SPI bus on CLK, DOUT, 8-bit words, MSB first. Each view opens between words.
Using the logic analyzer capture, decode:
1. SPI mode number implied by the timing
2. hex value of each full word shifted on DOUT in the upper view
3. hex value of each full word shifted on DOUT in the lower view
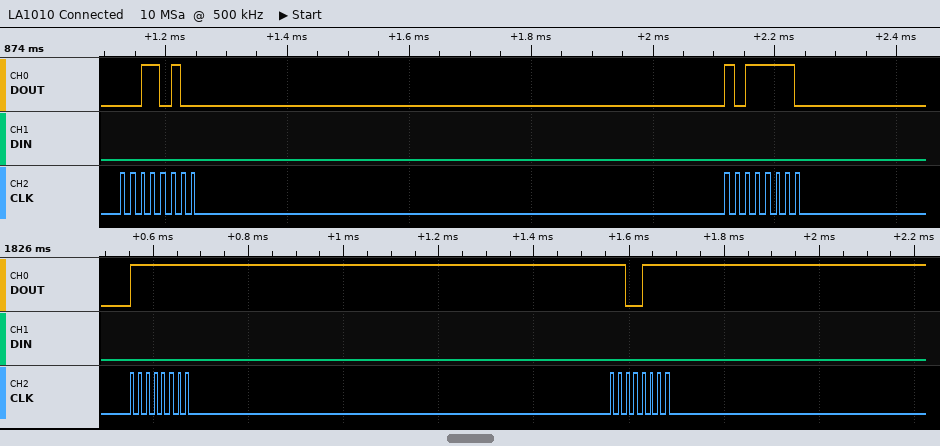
1
34, BE
FF, CF
